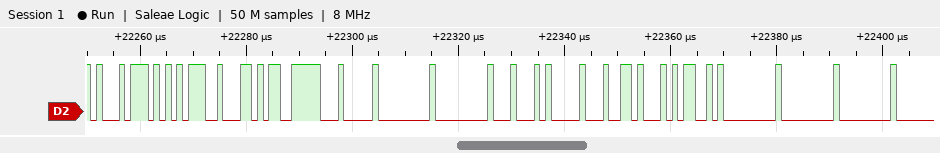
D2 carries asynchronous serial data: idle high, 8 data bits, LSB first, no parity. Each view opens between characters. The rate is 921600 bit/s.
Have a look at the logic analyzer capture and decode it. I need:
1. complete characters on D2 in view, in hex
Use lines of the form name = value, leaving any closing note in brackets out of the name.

complete characters on D2 in view, in hex = D1, D5, 62, F3, 04, 00, 00, 44, 10, 16, 4D, 00, 00, 00
